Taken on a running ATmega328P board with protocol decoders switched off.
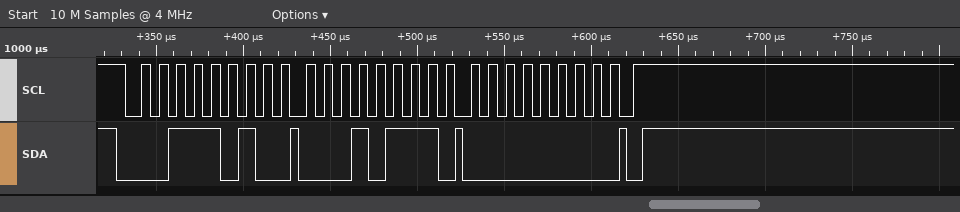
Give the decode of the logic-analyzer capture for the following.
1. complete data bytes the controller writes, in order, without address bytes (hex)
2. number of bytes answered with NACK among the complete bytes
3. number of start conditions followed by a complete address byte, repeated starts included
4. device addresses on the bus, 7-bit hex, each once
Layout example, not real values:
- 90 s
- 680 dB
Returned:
- 17 00
- 0
- 1
- 0x1D
